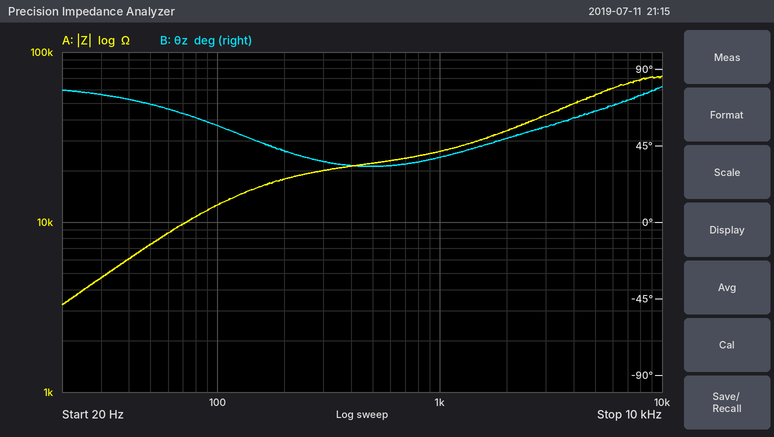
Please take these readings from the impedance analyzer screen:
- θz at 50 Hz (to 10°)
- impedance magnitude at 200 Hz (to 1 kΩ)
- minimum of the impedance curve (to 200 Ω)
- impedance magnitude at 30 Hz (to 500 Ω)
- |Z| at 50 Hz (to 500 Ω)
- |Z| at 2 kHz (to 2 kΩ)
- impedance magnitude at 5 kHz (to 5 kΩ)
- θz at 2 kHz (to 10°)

70°
18 kΩ
3.2 kΩ
4.5 kΩ
7.5 kΩ
34 kΩ
55 kΩ
50°
